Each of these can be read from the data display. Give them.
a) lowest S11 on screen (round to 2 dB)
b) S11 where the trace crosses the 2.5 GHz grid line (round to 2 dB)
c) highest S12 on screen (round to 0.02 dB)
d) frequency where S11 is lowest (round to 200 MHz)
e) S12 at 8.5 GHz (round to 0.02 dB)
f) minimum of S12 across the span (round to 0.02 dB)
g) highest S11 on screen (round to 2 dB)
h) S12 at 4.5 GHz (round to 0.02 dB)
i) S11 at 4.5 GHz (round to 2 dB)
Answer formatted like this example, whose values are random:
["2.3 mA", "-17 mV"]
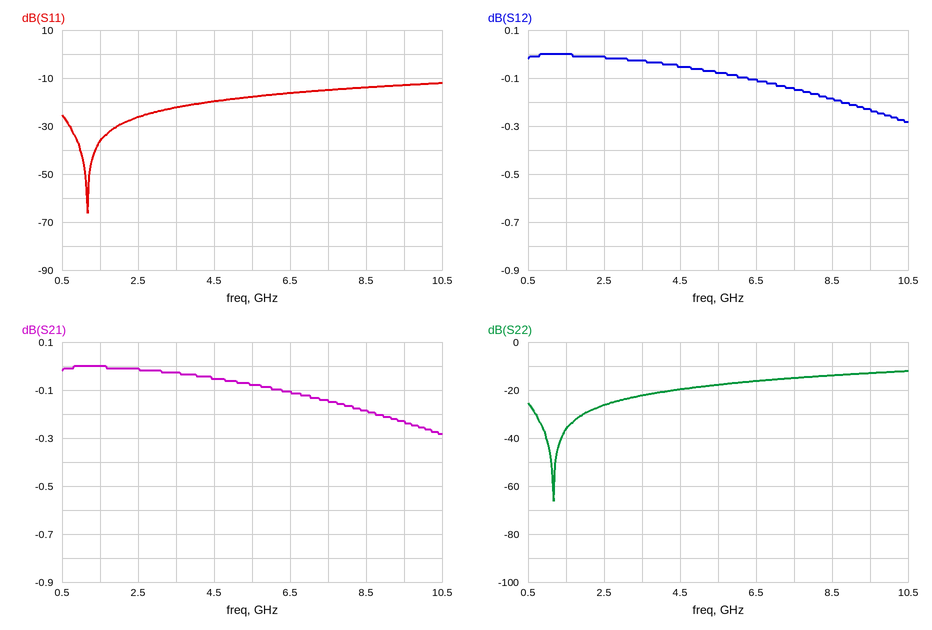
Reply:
["-66 dB", "-26 dB", "0.00 dB", "1.2 GHz", "-0.18 dB", "-0.28 dB", "-12 dB", "-0.06 dB", "-20 dB"]
